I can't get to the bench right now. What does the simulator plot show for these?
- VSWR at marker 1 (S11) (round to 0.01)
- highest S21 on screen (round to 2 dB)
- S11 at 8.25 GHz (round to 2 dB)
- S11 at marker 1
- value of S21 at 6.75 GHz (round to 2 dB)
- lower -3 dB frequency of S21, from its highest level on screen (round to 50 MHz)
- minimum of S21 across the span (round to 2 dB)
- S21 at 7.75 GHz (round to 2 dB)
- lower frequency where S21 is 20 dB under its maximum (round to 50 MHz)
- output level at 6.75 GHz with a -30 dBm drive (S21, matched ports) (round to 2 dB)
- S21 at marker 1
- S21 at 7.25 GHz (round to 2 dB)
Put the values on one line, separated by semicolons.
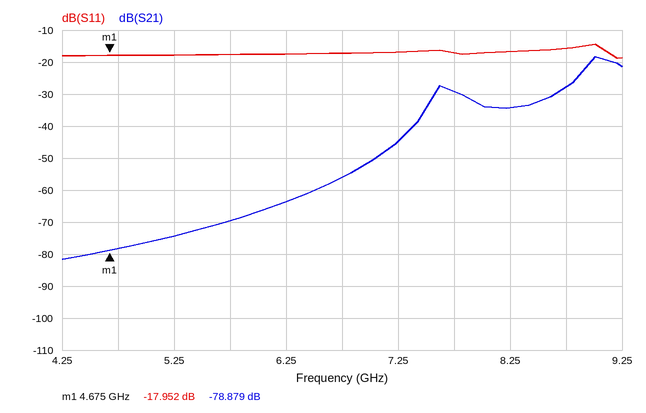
1.29; -18 dB; -16 dB; -17.952 dB; -56 dB; 8.95 GHz; -82 dB; -30 dB; 7.45 GHz; -86 dBm; -78.879 dB; -44 dB
